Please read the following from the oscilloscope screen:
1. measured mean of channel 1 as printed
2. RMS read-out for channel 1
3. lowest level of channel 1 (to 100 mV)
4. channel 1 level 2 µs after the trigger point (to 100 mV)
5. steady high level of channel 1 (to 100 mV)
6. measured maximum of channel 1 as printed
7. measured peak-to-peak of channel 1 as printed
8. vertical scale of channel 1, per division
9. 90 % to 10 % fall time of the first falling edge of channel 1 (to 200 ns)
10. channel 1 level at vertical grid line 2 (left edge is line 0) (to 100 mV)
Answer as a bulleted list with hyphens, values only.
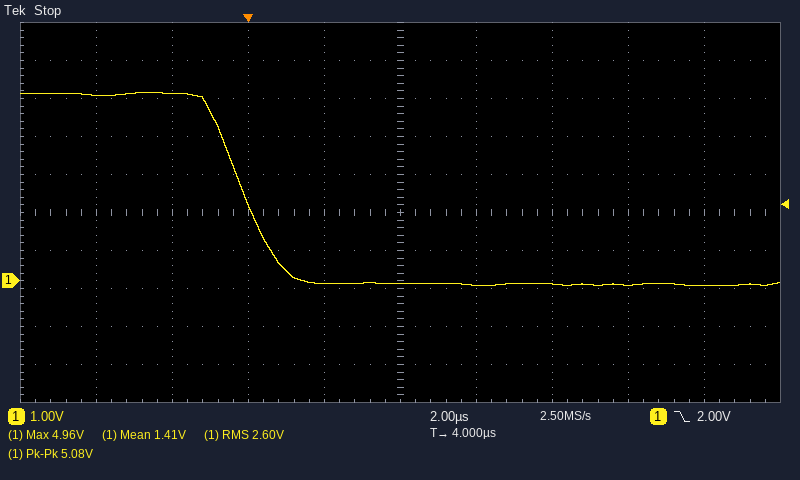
- 1.41 V
- 2.60 V
- -100 mV
- -100 mV
- 4.9 V
- 4.96 V
- 5.08 V
- 1 V
- 1.8 µs
- 4.9 V
